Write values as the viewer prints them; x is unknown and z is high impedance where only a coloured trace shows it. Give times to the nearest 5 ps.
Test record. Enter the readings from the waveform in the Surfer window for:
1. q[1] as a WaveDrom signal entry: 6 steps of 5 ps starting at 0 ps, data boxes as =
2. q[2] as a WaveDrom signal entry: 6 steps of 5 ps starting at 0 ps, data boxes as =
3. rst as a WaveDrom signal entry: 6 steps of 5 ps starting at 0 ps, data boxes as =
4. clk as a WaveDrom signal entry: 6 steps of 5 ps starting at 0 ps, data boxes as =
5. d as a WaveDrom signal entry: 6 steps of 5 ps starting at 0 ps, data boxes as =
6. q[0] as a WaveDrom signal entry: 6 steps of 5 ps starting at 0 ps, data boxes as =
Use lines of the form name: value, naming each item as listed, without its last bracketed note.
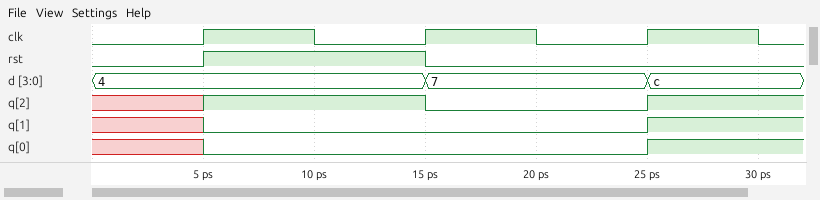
q[1] as a WaveDrom signal entry: 6 steps of 5 ps starting at 0 ps, data boxes as =: {name: 'q[1]', wave: 'x0...1'}
q[2] as a WaveDrom signal entry: 6 steps of 5 ps starting at 0 ps, data boxes as =: {name: 'q[2]', wave: 'x1.0.1'}
rst as a WaveDrom signal entry: 6 steps of 5 ps starting at 0 ps, data boxes as =: {name: 'rst', wave: '01.0..'}
clk as a WaveDrom signal entry: 6 steps of 5 ps starting at 0 ps, data boxes as =: {name: 'clk', wave: '010101'}
d as a WaveDrom signal entry: 6 steps of 5 ps starting at 0 ps, data boxes as =: {name: 'd', wave: '=..=.=', data: '4 7 c'}
q[0] as a WaveDrom signal entry: 6 steps of 5 ps starting at 0 ps, data boxes as =: {name: 'q[0]', wave: 'x0...1'}
